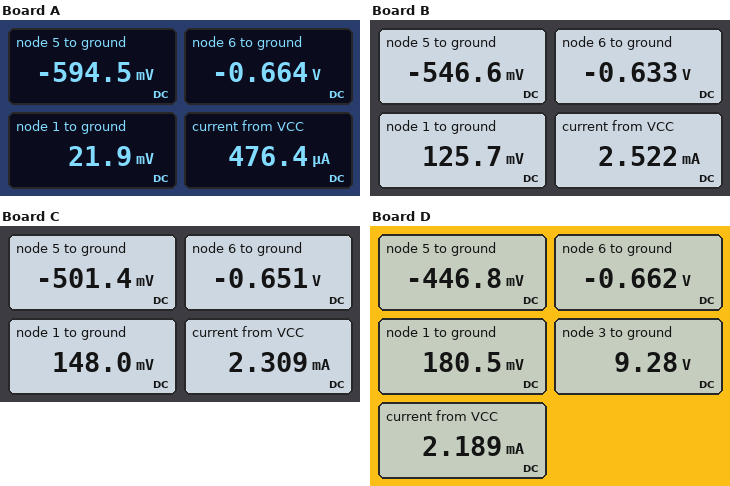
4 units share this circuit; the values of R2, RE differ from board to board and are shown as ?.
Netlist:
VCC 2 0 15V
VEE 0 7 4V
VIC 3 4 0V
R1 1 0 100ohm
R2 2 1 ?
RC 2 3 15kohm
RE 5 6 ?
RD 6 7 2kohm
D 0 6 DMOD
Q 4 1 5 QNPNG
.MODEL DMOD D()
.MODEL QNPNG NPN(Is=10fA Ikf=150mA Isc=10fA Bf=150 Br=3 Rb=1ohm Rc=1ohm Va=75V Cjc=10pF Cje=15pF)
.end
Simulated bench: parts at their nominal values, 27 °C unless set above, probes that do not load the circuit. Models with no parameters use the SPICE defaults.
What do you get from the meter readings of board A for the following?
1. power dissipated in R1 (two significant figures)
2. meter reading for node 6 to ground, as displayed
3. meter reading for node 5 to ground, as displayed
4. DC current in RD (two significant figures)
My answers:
4.8 µW
-0.664 V
-594.5 mV
1.7 mA
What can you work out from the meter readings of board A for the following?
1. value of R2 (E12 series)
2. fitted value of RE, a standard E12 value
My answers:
68 kΩ
270 Ω
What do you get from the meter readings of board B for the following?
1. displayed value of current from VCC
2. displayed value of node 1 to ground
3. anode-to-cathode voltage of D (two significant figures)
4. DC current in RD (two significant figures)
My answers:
2.522 mA
125.7 mV
630 mV
1.7 mA
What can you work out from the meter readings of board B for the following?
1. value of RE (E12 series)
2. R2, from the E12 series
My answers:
68 Ω
10 kΩ
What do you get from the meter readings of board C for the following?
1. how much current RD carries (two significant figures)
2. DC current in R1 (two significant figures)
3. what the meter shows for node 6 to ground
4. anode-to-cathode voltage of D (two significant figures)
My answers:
1.7 mA
1.5 mA
-0.651 V
650 mV
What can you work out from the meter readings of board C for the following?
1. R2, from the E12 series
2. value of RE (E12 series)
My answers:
10 kΩ
180 Ω
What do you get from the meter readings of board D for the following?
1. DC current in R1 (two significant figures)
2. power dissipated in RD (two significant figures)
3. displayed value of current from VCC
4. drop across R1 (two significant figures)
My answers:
1.8 mA
5.6 mW
2.189 mA
180 mV
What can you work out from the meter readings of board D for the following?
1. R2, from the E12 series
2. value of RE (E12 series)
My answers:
8.2 kΩ
560 Ω
